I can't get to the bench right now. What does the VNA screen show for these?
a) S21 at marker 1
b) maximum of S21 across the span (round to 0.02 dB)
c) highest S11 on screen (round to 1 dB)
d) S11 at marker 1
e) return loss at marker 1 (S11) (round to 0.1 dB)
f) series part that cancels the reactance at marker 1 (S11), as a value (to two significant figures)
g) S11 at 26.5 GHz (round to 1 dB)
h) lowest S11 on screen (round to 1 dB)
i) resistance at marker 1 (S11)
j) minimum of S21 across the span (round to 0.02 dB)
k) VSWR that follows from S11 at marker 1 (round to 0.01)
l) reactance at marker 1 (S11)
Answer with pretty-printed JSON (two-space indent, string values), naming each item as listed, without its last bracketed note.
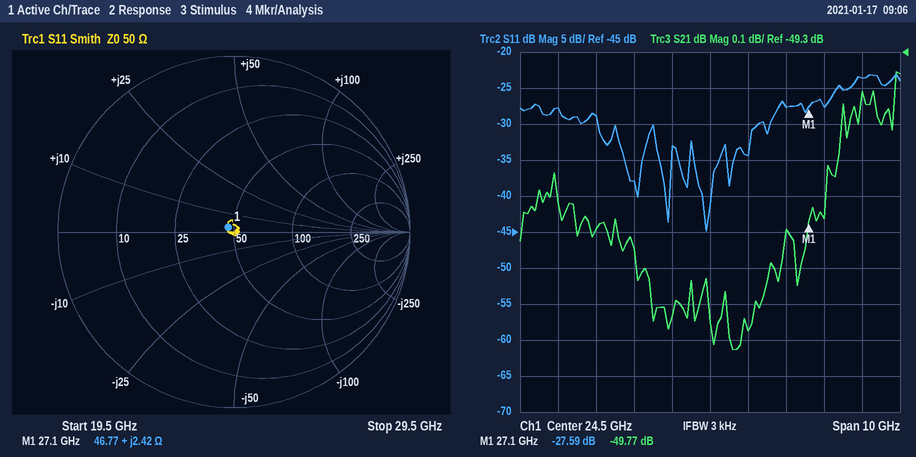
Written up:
{
  "S21 at marker 1": "-49.77 dB",
  "maximum of S21 across the span": "-49.36 dB",
  "highest S11 on screen": "-23 dB",
  "S11 at marker 1": "-27.59 dB",
  "return loss at marker 1 (S11)": "27.6 dB",
  "series part that cancels the reactance at marker 1 (S11), as a value": "2.4 pF",
  "S11 at 26.5 GHz": "-28 dB",
  "lowest S11 on screen": "-45 dB",
  "resistance at marker 1": "46.77 Ω",
  "minimum of S21 across the span": "-50.12 dB",
  "VSWR that follows from S11 at marker 1": "1.09",
  "reactance at marker 1": "+2.42 Ω"
}
